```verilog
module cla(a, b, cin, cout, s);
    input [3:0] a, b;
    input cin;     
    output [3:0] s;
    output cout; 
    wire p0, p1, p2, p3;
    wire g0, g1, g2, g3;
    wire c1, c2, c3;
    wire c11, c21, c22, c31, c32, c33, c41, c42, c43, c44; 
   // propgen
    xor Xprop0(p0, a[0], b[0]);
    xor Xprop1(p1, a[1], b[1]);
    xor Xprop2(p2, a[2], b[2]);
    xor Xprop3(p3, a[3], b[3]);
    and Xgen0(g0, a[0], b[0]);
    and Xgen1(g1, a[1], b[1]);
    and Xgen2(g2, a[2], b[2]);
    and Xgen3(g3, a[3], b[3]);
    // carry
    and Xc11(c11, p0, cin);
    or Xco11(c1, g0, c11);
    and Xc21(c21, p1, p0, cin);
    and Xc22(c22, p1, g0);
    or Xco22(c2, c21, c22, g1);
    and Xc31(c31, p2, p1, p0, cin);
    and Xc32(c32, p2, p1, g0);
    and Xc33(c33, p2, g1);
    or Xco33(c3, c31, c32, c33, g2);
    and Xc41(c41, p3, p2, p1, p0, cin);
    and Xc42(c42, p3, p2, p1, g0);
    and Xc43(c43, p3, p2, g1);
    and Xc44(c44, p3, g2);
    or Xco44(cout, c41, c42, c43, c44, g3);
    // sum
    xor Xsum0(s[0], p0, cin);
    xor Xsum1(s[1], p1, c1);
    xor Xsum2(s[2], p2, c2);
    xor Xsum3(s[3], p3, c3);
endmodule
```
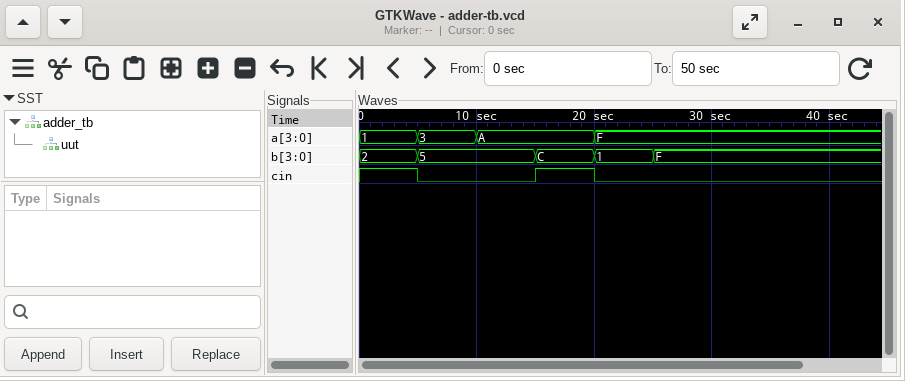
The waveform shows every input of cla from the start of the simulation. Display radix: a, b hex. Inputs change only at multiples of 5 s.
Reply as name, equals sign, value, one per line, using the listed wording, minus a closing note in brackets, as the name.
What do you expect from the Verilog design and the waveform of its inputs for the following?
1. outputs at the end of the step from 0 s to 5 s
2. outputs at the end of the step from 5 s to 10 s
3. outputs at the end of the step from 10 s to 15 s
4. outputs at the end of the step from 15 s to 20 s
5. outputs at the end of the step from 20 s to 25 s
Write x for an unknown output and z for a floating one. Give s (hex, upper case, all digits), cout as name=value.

outputs at the end of the step from 0 s to 5 s = s=4, cout=0
outputs at the end of the step from 5 s to 10 s = s=8, cout=0
outputs at the end of the step from 10 s to 15 s = s=F, cout=0
outputs at the end of the step from 15 s to 20 s = s=7, cout=1
outputs at the end of the step from 20 s to 25 s = s=0, cout=1
